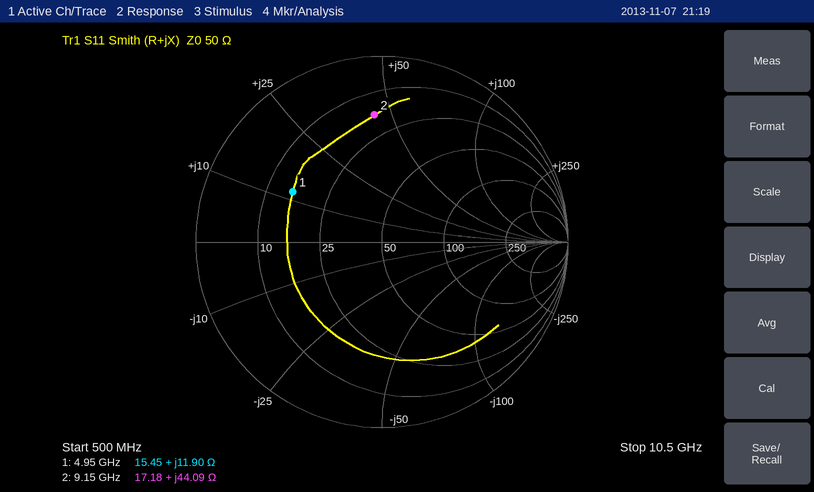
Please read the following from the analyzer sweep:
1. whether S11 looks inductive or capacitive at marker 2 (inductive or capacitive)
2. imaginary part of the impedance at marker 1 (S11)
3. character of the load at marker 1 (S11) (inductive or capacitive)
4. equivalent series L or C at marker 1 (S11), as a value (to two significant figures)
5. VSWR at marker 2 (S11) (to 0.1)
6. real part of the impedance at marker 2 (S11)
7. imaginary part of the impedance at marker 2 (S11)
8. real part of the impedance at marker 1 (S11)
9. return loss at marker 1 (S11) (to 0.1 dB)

inductive
+11.90 Ω
inductive
380 pH
5.3
17.18 Ω
+44.09 Ω
15.45 Ω
5.2 dB
